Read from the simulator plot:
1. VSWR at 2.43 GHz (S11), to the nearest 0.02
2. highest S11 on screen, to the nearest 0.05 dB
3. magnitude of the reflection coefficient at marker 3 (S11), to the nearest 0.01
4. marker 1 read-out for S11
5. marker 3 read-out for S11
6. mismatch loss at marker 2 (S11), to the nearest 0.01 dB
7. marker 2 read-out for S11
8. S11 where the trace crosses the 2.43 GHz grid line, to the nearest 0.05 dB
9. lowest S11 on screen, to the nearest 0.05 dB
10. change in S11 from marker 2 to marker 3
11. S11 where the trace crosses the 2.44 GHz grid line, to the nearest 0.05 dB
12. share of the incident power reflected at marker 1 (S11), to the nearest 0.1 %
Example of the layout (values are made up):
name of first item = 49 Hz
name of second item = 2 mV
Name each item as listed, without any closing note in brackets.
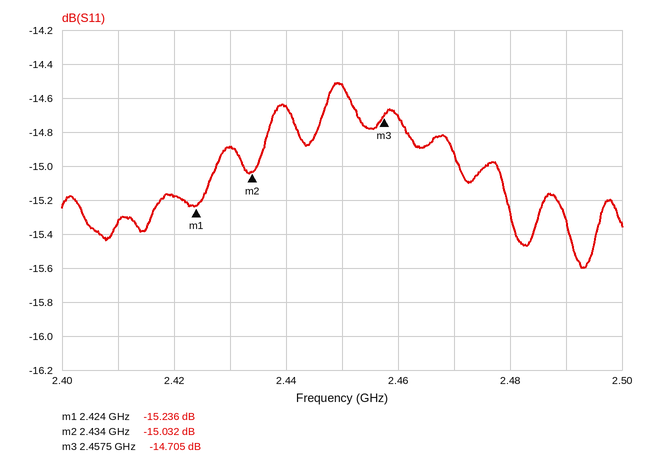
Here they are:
VSWR at 2.43 GHz (S11), to the nearest 0.02 = 1.44
highest S11 on screen, to the nearest 0.05 dB = -14.50 dB
magnitude of the reflection coefficient at marker 3 (S11), to the nearest 0.01 = 0.18
marker 1 read-out for S11 = -15.236 dB
marker 3 read-out for S11 = -14.705 dB
mismatch loss at marker 2 (S11), to the nearest 0.01 dB = 0.14 dB
marker 2 read-out for S11 = -15.032 dB
S11 where the trace crosses the 2.43 GHz grid line, to the nearest 0.05 dB = -14.90 dB
lowest S11 on screen, to the nearest 0.05 dB = -15.60 dB
change in S11 from marker 2 to marker 3 = 0.327 dB
S11 where the trace crosses the 2.44 GHz grid line, to the nearest 0.05 dB = -14.65 dB
share of the incident power reflected at marker 1 (S11), to the nearest 0.1 % = 3.0 %
